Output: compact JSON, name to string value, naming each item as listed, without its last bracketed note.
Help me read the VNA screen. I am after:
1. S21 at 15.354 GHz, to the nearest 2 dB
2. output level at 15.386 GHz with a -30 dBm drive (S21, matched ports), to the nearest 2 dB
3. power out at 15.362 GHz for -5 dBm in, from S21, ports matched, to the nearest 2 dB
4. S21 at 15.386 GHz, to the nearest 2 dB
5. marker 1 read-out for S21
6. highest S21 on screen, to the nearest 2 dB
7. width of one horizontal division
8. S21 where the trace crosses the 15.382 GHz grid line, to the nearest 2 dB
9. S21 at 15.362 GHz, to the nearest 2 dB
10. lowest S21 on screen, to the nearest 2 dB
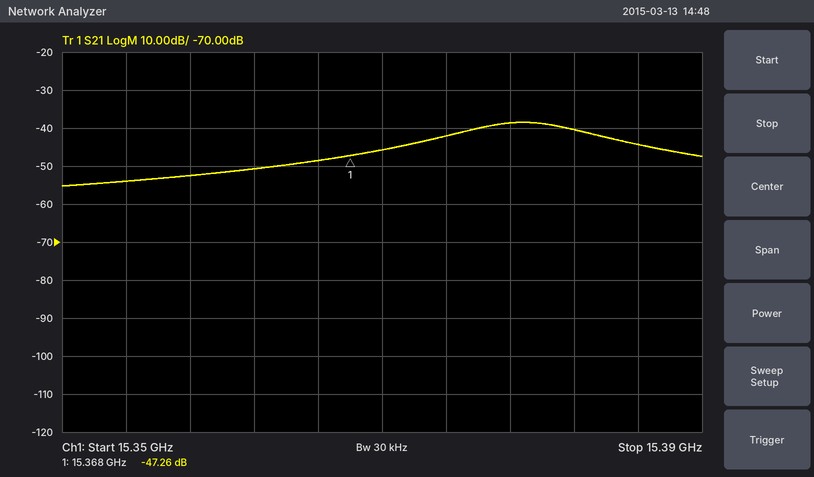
{"S21 at 15.354 GHz, to the nearest 2 dB": "-54 dB", "output level at 15.386 GHz with a -30 dBm drive (S21, matched ports), to the nearest 2 dB": "-74 dBm", "power out at 15.362 GHz for -5 dBm in, from S21, ports matched, to the nearest 2 dB": "-56 dBm", "S21 at 15.386 GHz, to the nearest 2 dB": "-44 dB", "marker 1 read-out for S21": "-47.26 dB", "highest S21 on screen, to the nearest 2 dB": "-38 dB", "width of one horizontal division": "4 MHz", "S21 where the trace crosses the 15.382 GHz grid line, to the nearest 2 dB": "-40 dB", "S21 at 15.362 GHz, to the nearest 2 dB": "-50 dB", "lowest S21 on screen, to the nearest 2 dB": "-56 dB"}
